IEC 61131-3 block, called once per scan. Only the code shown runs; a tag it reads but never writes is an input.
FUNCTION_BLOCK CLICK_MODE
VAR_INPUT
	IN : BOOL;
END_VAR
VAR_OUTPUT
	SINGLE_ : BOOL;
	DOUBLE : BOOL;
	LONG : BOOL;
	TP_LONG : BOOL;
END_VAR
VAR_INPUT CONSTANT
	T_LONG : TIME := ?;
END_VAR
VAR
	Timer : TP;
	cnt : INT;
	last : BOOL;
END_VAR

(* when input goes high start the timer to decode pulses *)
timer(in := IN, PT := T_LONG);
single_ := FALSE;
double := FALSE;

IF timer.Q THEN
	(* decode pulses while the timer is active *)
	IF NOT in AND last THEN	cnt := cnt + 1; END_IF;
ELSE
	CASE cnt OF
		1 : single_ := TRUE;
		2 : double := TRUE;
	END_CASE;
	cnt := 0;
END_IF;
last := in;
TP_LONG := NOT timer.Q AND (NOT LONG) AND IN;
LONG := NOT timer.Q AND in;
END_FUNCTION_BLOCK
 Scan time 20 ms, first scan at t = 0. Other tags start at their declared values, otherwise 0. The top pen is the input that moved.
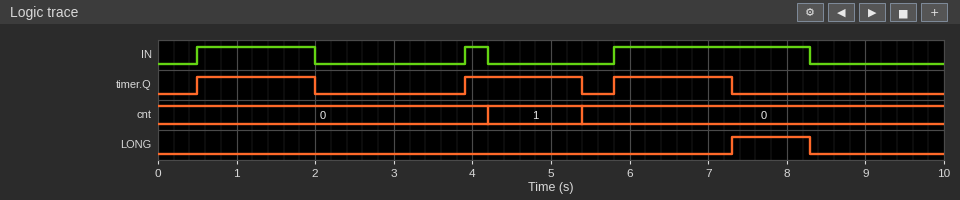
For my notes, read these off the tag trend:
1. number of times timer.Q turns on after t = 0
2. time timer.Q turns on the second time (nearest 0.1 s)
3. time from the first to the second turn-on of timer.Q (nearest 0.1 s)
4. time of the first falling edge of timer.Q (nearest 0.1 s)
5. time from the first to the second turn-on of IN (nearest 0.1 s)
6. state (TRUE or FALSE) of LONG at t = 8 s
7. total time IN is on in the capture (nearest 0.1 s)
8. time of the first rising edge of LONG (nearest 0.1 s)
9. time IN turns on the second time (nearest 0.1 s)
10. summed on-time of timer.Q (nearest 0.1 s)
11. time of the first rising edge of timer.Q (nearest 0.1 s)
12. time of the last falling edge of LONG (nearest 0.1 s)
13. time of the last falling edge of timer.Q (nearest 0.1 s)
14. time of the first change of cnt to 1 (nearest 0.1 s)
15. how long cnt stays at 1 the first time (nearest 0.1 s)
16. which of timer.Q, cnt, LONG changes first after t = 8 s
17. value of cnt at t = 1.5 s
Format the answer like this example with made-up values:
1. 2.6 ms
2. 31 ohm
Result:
1. 3
2. 3.9 s
3. 3.4 s
4. 2.0 s
5. 3.4 s
6. TRUE
7. 4.3 s
8. 7.3 s
9. 3.9 s
10. 4.5 s
11. 0.5 s
12. 8.3 s
13. 7.3 s
14. 4.2 s
15. 1.2 s
16. LONG
17. 0
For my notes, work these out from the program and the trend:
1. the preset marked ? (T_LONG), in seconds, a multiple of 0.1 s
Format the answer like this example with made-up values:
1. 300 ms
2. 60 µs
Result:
1. 1.5 s
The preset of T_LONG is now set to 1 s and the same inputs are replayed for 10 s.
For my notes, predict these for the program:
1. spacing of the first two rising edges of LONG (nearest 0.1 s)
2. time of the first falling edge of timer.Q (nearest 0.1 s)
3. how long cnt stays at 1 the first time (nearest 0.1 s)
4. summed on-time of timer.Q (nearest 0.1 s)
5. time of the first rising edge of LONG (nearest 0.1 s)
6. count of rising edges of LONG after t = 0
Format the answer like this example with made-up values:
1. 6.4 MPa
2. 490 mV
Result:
1. 5.3 s
2. 1.5 s
3. 0.7 s
4. 3.0 s
5. 1.5 s
6. 2
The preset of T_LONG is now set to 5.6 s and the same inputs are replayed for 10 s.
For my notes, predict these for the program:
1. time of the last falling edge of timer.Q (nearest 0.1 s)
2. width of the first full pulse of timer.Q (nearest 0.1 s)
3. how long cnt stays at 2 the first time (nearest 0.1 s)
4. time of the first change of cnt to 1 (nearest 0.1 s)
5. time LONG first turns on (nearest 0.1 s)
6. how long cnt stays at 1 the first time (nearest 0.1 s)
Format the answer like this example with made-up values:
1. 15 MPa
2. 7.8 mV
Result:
1. 6.1 s
2. 5.6 s
3. 1.9 s
4. 2.0 s
5. 6.1 s
6. 2.2 s
